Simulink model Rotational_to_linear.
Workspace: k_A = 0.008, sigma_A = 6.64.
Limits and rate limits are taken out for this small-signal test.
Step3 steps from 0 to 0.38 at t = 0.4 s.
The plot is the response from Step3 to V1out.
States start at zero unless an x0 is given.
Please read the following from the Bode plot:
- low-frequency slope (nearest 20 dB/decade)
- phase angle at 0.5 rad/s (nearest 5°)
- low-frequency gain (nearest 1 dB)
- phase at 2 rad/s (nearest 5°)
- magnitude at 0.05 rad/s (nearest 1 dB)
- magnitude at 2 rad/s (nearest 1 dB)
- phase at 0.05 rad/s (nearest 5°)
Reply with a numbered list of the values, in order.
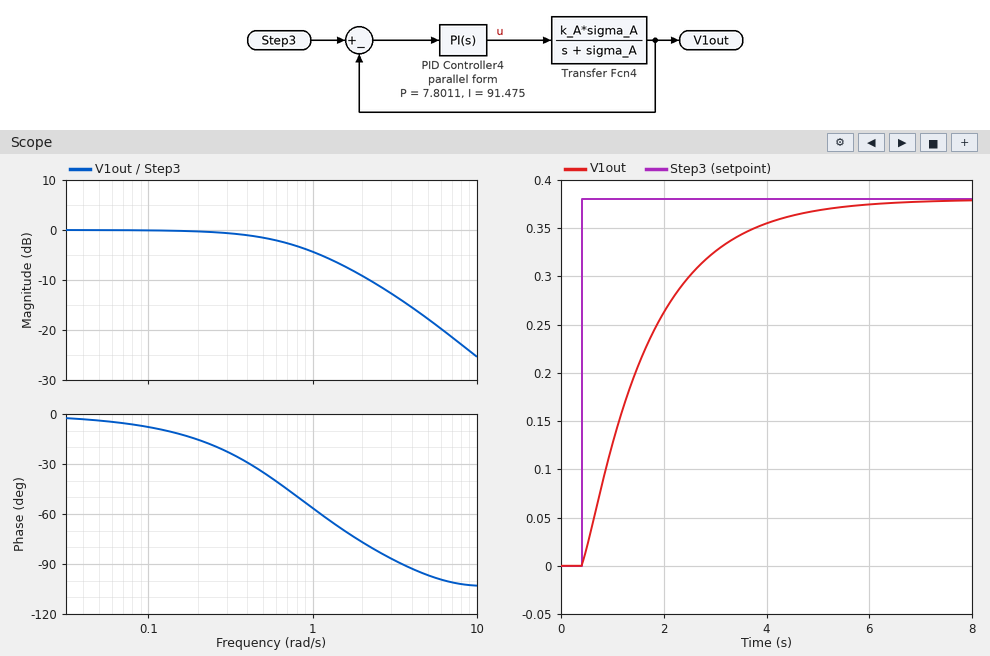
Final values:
1. 0 dB/decade
2. -35°
3. 0 dB
4. -75°
5. 0 dB
6. -9 dB
7. -5°
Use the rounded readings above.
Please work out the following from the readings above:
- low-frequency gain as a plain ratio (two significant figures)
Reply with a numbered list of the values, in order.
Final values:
1. 1.0
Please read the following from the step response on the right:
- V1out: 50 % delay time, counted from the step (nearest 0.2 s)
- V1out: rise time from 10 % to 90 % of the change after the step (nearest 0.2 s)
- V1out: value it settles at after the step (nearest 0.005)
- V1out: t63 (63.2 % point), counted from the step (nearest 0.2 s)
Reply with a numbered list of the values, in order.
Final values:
1. 1.0 s
2. 2.8 s
3. 0.380
4. 1.4 s
